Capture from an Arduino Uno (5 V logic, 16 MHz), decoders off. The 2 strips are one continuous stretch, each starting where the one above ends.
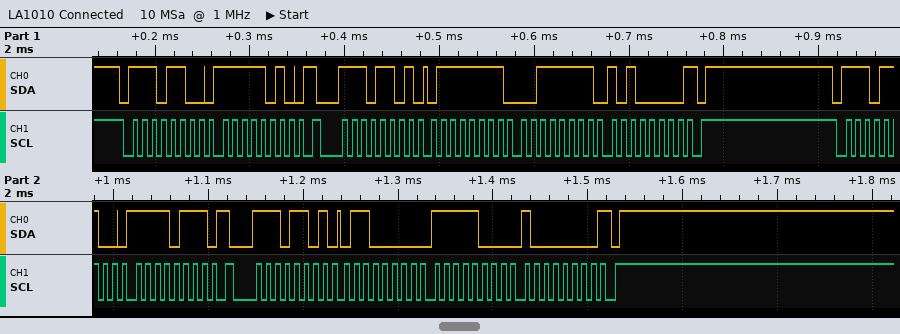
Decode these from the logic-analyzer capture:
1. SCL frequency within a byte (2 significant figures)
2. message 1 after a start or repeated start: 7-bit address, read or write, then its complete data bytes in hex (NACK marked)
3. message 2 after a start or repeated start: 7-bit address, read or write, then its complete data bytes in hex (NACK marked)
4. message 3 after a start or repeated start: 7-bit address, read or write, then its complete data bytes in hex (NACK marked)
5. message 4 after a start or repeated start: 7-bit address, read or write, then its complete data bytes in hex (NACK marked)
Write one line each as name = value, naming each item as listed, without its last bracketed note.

SCL frequency within a byte = 100 kHz
message 1 after a start or repeated start: 7-bit address, read or write, then its complete data bytes in hex = 0x76 write: FA
message 2 after a start or repeated start: 7-bit address, read or write, then its complete data bytes in hex = 0x76 read: 7F 3F A0 NACK
message 3 after a start or repeated start: 7-bit address, read or write, then its complete data bytes in hex = 0x76 write: F7
message 4 after a start or repeated start: 7-bit address, read or write, then its complete data bytes in hex = 0x76 read: 60 F8 80 NACK
